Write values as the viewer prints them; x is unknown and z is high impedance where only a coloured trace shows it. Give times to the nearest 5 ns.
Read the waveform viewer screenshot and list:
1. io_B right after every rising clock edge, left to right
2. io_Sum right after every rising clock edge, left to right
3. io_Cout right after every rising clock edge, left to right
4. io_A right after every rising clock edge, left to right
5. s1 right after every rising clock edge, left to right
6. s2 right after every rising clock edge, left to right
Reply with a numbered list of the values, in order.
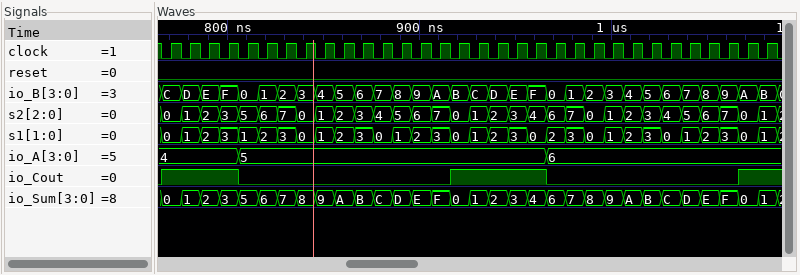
1. C, D, E, F, 0, 1, 2, 3, 4, 5, 6, 7, 8, 9, A, B, C, D, E, F, 0, 1, 2, 3, 4, 5, 6, 7, 8, 9, A, B
2. 0, 1, 2, 3, 5, 6, 7, 8, 9, A, B, C, D, E, F, 0, 1, 2, 3, 4, 6, 7, 8, 9, A, B, C, D, E, F, 0, 1
3. 1 1 1 1 0 0 0 0 0 0 0 0 0 0 0 1 1 1 1 1 0 0 0 0 0 0 0 0 0 0 1 1
4. 4, 4, 4, 4, 5, 5, 5, 5, 5, 5, 5, 5, 5, 5, 5, 5, 5, 5, 5, 5, 6, 6, 6, 6, 6, 6, 6, 6, 6, 6, 6, 6
5. 0, 1, 2, 3, 1, 2, 3, 0, 1, 2, 3, 0, 1, 2, 3, 0, 1, 2, 3, 0, 2, 3, 0, 1, 2, 3, 0, 1, 2, 3, 0, 1
6. 0, 1, 2, 3, 5, 6, 7, 0, 1, 2, 3, 4, 5, 6, 7, 0, 1, 2, 3, 4, 6, 7, 0, 1, 2, 3, 4, 5, 6, 7, 0, 1
